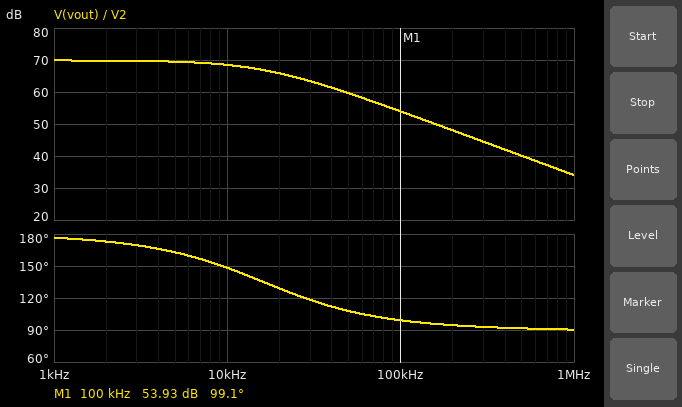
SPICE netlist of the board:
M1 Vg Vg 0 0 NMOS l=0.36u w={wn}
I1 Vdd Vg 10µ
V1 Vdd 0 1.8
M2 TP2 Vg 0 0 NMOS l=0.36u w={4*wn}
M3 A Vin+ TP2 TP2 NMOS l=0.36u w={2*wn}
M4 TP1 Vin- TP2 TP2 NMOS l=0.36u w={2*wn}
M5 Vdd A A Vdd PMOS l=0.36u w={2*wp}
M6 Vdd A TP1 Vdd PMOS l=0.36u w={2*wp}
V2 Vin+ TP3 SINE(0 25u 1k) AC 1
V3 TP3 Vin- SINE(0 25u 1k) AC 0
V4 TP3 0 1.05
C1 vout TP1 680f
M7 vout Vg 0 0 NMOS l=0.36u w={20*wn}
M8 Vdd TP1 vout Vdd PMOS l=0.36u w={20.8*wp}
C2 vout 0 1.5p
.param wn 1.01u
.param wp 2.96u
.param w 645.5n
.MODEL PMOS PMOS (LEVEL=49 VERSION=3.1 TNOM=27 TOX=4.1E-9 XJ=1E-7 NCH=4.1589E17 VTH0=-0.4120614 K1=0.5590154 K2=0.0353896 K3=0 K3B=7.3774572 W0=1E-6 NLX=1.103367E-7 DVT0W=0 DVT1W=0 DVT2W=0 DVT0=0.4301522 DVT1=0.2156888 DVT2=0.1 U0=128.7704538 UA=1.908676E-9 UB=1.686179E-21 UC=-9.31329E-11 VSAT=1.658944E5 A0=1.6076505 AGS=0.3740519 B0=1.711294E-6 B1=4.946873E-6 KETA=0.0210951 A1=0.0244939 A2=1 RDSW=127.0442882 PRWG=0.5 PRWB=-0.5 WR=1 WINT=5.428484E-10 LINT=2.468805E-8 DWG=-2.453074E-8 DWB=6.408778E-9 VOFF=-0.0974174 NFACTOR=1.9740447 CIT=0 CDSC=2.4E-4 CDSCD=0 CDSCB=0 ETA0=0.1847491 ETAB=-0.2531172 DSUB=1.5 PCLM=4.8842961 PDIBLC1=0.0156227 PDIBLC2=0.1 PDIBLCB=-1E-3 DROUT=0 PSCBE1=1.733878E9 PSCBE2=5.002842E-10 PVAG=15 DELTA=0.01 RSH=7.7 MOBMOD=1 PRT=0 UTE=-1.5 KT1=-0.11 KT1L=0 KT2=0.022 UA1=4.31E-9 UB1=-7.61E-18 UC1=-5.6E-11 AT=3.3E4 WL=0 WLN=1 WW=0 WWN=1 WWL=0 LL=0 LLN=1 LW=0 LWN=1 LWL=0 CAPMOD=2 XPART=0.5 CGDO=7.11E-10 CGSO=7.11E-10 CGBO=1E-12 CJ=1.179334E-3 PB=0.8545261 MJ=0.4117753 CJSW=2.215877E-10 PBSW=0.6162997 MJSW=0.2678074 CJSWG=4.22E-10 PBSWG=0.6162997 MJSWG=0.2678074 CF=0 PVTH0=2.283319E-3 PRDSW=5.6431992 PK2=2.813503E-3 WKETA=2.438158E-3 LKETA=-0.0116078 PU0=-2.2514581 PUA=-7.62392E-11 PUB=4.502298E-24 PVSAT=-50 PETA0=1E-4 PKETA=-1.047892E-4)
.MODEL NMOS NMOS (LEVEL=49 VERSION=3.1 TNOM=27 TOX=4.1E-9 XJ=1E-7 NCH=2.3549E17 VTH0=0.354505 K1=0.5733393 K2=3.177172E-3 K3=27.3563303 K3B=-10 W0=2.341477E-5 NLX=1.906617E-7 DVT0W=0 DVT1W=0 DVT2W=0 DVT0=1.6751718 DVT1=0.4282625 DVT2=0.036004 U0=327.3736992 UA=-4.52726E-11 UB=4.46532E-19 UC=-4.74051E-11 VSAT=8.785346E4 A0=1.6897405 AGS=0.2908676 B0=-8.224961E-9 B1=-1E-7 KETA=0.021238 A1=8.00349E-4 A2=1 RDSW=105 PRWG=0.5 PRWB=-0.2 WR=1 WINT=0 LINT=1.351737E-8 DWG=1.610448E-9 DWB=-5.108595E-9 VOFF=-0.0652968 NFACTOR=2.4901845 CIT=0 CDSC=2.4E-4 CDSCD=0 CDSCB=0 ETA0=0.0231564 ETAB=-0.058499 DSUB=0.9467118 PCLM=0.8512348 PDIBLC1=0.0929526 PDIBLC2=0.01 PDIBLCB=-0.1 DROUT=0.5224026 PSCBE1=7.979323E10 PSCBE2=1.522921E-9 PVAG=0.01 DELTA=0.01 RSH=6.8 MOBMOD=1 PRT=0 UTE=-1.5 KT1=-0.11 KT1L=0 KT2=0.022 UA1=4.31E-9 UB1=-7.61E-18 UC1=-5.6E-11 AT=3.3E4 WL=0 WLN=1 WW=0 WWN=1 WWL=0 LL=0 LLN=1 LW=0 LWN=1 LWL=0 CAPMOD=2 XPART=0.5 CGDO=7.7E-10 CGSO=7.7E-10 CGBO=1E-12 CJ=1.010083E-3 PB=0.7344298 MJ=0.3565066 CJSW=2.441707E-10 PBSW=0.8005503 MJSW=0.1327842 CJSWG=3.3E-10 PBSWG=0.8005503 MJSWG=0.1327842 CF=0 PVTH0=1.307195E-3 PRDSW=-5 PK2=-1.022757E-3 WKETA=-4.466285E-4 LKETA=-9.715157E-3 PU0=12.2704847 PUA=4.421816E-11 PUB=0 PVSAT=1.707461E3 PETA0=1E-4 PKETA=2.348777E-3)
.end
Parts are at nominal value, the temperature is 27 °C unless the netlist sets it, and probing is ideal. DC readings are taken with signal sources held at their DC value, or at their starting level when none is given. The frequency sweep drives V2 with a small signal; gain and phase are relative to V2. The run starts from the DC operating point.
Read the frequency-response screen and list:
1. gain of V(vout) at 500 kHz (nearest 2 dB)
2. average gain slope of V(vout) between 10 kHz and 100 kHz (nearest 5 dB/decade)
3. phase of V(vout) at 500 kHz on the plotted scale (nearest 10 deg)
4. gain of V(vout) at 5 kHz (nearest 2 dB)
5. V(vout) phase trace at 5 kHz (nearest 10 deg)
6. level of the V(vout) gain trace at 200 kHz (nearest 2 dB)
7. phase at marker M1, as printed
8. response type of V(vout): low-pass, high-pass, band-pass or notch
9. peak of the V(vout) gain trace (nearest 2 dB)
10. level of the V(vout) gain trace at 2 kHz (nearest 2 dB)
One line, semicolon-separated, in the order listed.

40 dB; -15 dB/decade; 90 deg; 70 dB; 160 deg; 48 dB; 99.1 deg; low-pass; 70 dB; 70 dB
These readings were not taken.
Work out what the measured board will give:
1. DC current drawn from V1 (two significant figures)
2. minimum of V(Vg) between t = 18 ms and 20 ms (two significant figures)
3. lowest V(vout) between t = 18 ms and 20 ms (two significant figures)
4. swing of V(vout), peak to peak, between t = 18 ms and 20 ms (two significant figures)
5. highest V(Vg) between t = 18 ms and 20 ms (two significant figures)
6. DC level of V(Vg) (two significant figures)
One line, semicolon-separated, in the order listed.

250 µA; 650 mV; 760 mV; 310 mV; 650 mV; 650 mV
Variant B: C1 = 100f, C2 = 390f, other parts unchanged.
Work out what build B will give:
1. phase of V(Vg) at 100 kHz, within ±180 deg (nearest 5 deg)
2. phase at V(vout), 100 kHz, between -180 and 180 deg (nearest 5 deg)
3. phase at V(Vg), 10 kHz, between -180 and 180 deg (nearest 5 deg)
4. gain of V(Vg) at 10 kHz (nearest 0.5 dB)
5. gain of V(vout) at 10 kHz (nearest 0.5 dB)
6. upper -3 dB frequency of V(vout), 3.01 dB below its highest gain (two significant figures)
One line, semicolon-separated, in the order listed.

-140 deg; 130 deg; -95 deg; -32.5 dB; 70.0 dB; 80 kHz
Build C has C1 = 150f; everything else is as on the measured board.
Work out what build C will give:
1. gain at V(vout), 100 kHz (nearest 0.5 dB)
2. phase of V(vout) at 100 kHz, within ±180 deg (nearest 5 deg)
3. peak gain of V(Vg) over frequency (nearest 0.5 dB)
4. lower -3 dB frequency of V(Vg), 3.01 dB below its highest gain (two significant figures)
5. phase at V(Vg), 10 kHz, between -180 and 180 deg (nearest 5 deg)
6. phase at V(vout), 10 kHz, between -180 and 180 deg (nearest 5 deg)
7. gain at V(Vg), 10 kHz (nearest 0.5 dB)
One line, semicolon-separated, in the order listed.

64.0 dB; 120 deg; -17.0 dB; 59 kHz; -100 deg; 170 deg; -32.5 dB
